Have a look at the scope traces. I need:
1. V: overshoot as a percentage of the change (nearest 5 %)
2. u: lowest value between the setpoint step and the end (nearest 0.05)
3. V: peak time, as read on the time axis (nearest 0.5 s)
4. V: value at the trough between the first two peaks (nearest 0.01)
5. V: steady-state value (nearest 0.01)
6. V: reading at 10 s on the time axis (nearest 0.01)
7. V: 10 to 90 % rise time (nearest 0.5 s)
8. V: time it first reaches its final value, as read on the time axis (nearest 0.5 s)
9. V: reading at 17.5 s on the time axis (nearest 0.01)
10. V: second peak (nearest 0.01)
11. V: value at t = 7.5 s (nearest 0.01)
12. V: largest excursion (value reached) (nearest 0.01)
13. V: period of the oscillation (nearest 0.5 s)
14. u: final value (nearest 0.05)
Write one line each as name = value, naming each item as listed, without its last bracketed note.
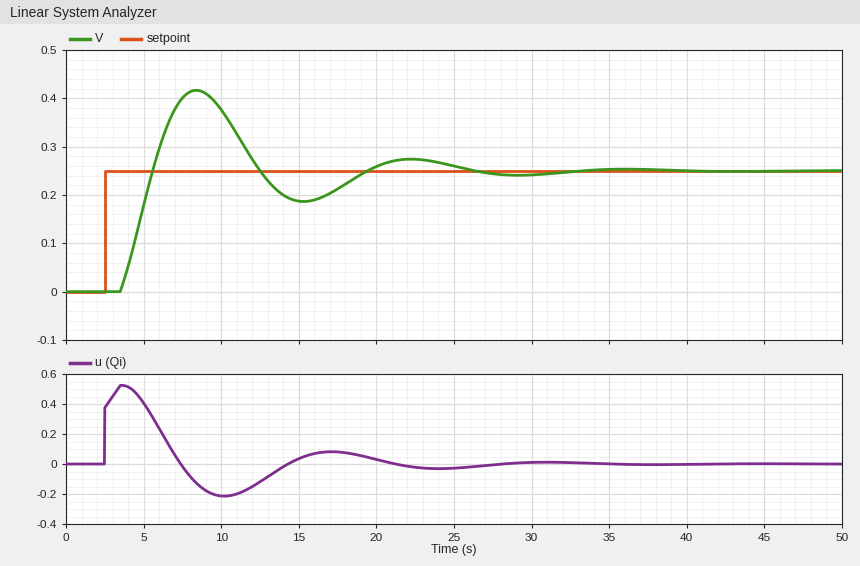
V: overshoot as a percentage of the change = 65 %
u: lowest value between the setpoint step and the end = -0.20
V: peak time, as read on the time axis = 8.5 s
V: value at the trough between the first two peaks = 0.19
V: steady-state value = 0.25
V: reading at 10 s on the time axis = 0.38
V: 10 to 90 % rise time = 1.5 s
V: time it first reaches its final value, as read on the time axis = 5.5 s
V: reading at 17.5 s on the time axis = 0.21
V: second peak = 0.27
V: value at t = 7.5 s = 0.40
V: largest excursion (value reached) = 0.42
V: period of the oscillation = 14.0 s
u: final value = 0.00
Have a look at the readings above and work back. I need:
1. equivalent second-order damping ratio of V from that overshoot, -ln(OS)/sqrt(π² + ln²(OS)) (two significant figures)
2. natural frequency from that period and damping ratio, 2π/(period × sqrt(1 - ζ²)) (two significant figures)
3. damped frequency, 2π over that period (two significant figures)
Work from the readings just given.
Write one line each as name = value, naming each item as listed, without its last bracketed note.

equivalent second-order damping ratio of V from that overshoot, -ln(OS)/sqrt(π² + ln²(OS)) = 0.14
natural frequency from that period and damping ratio, 2π/(period × sqrt(1 - ζ²)) = 0.45 rad/s
damped frequency, 2π over that period = 0.45 rad/s
